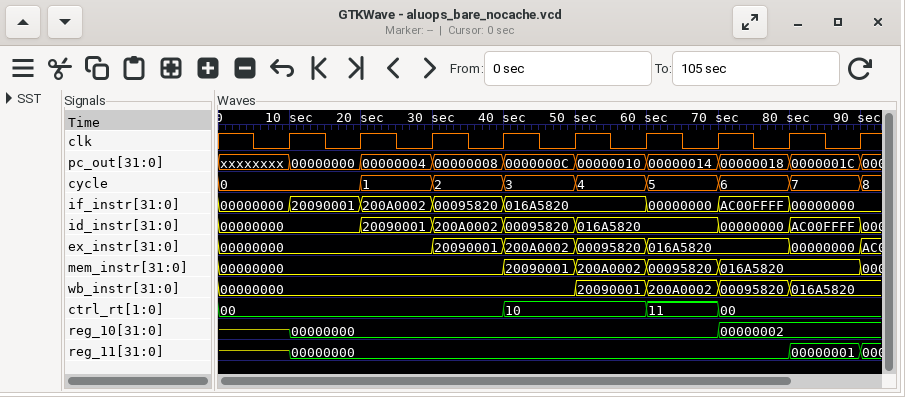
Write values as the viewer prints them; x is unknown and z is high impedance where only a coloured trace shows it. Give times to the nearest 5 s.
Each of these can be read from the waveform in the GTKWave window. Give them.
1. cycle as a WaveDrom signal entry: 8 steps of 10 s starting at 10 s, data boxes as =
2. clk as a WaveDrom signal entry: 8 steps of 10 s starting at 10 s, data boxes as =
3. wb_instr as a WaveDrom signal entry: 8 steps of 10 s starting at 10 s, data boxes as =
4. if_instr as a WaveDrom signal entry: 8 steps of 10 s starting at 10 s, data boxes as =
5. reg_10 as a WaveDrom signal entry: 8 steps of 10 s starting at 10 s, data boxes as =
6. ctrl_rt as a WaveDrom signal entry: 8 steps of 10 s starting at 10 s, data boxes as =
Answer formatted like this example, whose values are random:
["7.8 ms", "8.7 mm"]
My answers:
["{name: 'cycle', wave: '========', data: '0 1 2 3 4 5 6 7'}", "{name: 'clk', wave: 'p.......'}", "{name: 'wb_instr', wave: '=...====', data: '00000000 20090001 200A0002 00095820 016A5820'}", "{name: 'if_instr', wave: '====.===', data: '20090001 200A0002 00095820 016A5820 00000000 AC00FFFF 00000000'}", "{name: 'reg_10', wave: '=.....=.', data: '00000000 00000002'}", "{name: 'ctrl_rt', wave: '=..=.==.', data: '00 10 11 00'}"]
